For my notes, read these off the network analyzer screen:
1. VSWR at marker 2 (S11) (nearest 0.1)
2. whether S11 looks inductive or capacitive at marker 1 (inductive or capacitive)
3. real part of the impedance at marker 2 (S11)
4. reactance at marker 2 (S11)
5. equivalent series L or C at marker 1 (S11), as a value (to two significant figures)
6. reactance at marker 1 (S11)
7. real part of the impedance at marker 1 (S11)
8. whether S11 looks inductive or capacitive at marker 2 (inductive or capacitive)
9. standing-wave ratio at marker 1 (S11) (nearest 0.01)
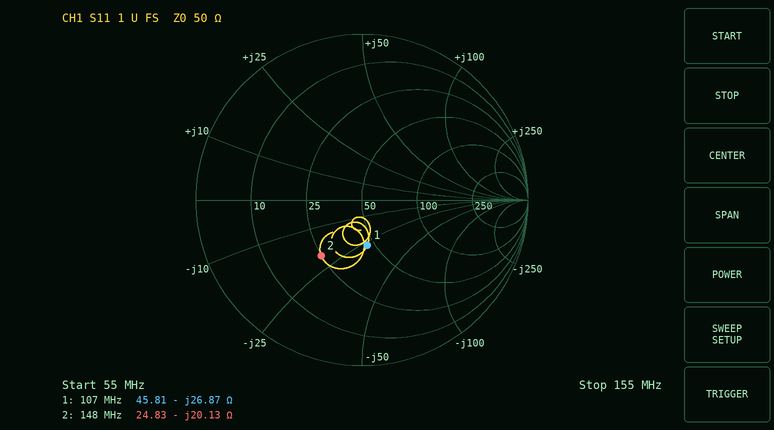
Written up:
2.4
capacitive
24.83 Ω
-20.13 Ω
55 pF
-26.87 Ω
45.81 Ω
capacitive
1.75
